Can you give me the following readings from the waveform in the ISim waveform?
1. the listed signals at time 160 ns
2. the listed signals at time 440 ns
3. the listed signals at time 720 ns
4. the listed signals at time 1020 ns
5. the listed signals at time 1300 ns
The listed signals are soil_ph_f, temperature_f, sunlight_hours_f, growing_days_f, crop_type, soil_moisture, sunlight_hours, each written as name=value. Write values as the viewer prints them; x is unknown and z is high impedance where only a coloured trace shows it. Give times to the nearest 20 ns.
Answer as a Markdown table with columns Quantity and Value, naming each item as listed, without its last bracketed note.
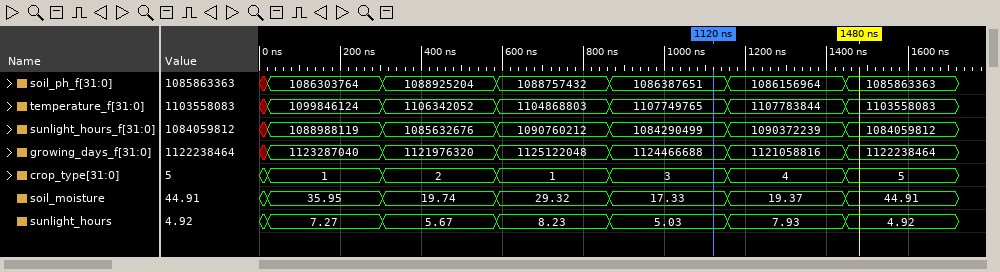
| Quantity | Value |
|---|---|
| the listed signals at time 160 ns | soil_ph_f=1086303764, temperature_f=1099846124, sunlight_hours_f=1088988119, growing_days_f=1123287040, crop_type=1, soil_moisture=35.95, sunlight_hours=7.27 |
| the listed signals at time 440 ns | soil_ph_f=1088925204, temperature_f=1106342052, sunlight_hours_f=1085632676, growing_days_f=1121976320, crop_type=2, soil_moisture=19.74, sunlight_hours=5.67 |
| the listed signals at time 720 ns | soil_ph_f=1088757432, temperature_f=1104868803, sunlight_hours_f=1090760212, growing_days_f=1125122048, crop_type=1, soil_moisture=29.32, sunlight_hours=8.23 |
| the listed signals at time 1020 ns | soil_ph_f=1086387651, temperature_f=1107749765, sunlight_hours_f=1084290499, growing_days_f=1124466688, crop_type=3, soil_moisture=17.33, sunlight_hours=5.03 |
| the listed signals at time 1300 ns | soil_ph_f=1086156964, temperature_f=1107783844, sunlight_hours_f=1090372239, growing_days_f=1121058816, crop_type=4, soil_moisture=19.37, sunlight_hours=7.93 |
